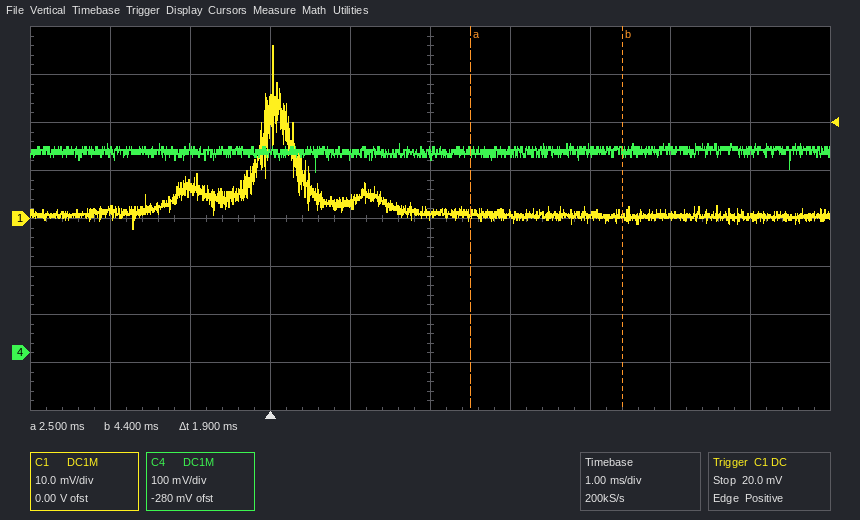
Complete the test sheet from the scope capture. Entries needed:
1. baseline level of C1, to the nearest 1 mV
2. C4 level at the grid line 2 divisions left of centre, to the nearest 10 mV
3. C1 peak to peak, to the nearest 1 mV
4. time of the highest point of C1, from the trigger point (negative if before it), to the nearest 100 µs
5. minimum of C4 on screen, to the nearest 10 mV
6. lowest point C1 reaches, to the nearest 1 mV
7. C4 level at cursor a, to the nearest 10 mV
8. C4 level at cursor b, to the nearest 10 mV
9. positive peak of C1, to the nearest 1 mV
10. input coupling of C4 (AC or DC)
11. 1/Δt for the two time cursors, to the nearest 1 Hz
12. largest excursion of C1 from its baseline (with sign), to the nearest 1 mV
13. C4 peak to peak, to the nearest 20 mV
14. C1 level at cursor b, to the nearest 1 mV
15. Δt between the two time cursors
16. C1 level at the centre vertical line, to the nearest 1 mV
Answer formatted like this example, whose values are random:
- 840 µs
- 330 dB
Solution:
- 1 mV
- 420 mV
- 38 mV
- 0.0 ms
- 380 mV
- -2 mV
- 420 mV
- 420 mV
- 36 mV
- DC
- 526 Hz
- +35 mV
- 60 mV
- 1 mV
- 1.9 ms
- 1 mV
